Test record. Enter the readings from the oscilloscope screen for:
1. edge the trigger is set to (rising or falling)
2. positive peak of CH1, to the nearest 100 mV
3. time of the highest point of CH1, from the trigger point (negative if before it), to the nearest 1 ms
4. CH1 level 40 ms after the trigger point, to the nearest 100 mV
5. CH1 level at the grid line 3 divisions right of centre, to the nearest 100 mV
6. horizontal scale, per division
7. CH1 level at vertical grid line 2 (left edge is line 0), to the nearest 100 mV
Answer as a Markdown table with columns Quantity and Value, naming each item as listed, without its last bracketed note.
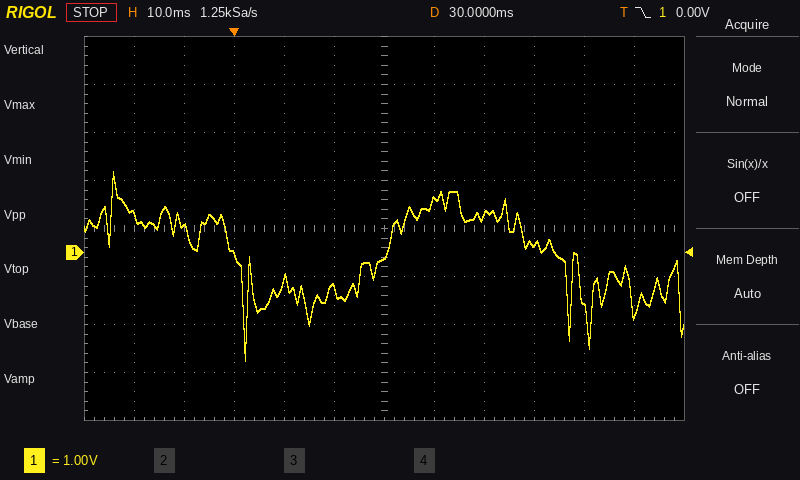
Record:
| Quantity | Value |
|---|---|
| edge the trigger is set to | falling |
| positive peak of CH1, to the nearest 100 mV | 1.7 V |
| time of the highest point of CH1, from the trigger point (negative if before it), to the nearest 1 ms | -24 ms |
| CH1 level 40 ms after the trigger point, to the nearest 100 mV | 1.1 V |
| CH1 level at the grid line 3 divisions right of centre, to the nearest 100 mV | 200 mV |
| horizontal scale, per division | 10 ms |
| CH1 level at vertical grid line 2 (left edge is line 0), to the nearest 100 mV | 500 mV |
